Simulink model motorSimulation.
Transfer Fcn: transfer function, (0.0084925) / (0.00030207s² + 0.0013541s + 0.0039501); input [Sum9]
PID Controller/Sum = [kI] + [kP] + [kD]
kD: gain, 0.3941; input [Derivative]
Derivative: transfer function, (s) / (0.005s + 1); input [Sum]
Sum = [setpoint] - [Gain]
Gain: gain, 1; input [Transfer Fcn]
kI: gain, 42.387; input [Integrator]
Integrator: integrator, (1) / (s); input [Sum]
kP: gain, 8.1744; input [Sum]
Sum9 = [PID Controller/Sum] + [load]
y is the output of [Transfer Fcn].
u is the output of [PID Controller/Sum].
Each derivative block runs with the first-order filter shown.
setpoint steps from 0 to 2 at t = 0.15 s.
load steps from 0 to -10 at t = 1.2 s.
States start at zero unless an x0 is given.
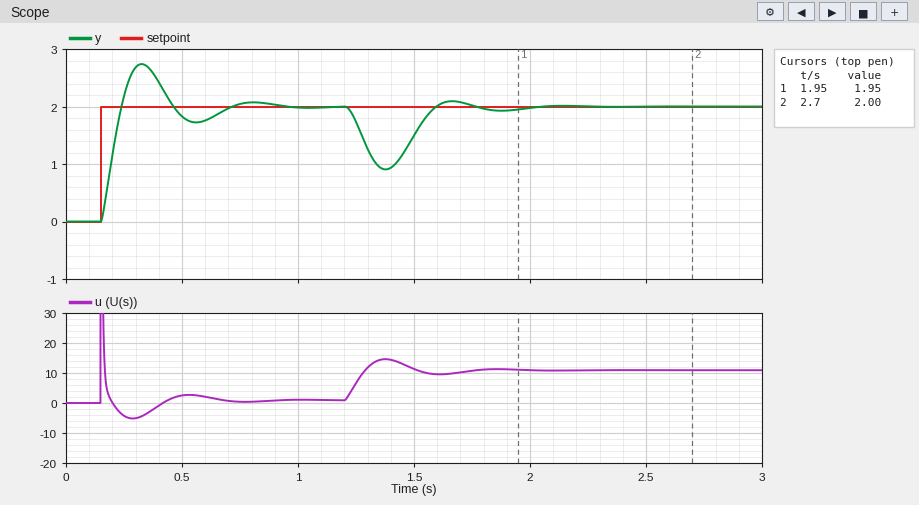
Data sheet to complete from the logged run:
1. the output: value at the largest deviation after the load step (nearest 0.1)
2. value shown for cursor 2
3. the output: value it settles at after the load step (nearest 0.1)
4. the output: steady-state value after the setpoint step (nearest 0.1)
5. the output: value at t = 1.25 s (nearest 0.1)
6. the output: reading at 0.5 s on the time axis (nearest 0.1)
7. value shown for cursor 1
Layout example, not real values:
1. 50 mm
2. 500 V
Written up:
1. 0.9
2. 2.00
3. 2.0
4. 2.0
5. 1.7
6. 1.8
7. 1.95
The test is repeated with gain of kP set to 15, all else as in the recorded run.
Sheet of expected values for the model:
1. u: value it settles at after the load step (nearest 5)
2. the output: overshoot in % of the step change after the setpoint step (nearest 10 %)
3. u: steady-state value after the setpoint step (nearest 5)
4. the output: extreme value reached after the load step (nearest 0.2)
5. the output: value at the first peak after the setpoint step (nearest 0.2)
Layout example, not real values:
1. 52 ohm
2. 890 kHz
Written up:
1. 10
2. 40 %
3. 0
4. 1.2
5. 2.8
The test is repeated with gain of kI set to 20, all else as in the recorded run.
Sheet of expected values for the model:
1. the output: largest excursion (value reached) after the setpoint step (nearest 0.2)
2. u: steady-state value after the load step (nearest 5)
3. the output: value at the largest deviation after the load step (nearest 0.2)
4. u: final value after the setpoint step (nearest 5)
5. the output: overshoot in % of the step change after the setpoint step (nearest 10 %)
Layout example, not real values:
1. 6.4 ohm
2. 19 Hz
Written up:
1. 2.6
2. 10
3. 0.8
4. 0
5. 30 %
